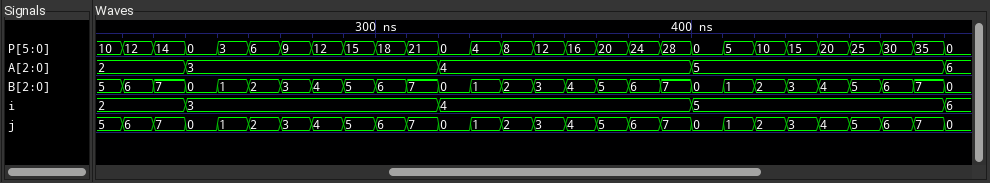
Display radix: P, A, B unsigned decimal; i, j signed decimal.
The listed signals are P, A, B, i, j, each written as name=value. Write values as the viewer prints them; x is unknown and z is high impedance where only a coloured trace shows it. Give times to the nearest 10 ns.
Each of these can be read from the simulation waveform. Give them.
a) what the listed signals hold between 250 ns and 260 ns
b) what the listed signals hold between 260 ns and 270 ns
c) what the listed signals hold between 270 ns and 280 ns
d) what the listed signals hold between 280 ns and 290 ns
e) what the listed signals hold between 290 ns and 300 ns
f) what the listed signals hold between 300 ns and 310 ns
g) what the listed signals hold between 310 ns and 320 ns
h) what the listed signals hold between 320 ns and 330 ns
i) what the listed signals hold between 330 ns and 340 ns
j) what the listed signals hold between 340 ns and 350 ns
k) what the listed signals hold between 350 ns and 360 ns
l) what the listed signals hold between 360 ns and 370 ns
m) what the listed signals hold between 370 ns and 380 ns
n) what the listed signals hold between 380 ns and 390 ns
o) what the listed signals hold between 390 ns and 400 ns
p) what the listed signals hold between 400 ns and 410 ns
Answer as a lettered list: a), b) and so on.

a) P=3, A=3, B=1, i=3, j=1
b) P=6, A=3, B=2, i=3, j=2
c) P=9, A=3, B=3, i=3, j=3
d) P=12, A=3, B=4, i=3, j=4
e) P=15, A=3, B=5, i=3, j=5
f) P=18, A=3, B=6, i=3, j=6
g) P=21, A=3, B=7, i=3, j=7
h) P=0, A=4, B=0, i=4, j=0
i) P=4, A=4, B=1, i=4, j=1
j) P=8, A=4, B=2, i=4, j=2
k) P=12, A=4, B=3, i=4, j=3
l) P=16, A=4, B=4, i=4, j=4
m) P=20, A=4, B=5, i=4, j=5
n) P=24, A=4, B=6, i=4, j=6
o) P=28, A=4, B=7, i=4, j=7
p) P=0, A=5, B=0, i=5, j=0
